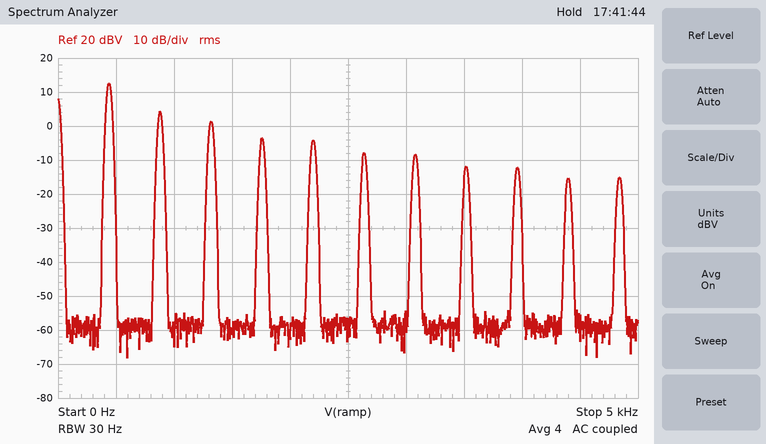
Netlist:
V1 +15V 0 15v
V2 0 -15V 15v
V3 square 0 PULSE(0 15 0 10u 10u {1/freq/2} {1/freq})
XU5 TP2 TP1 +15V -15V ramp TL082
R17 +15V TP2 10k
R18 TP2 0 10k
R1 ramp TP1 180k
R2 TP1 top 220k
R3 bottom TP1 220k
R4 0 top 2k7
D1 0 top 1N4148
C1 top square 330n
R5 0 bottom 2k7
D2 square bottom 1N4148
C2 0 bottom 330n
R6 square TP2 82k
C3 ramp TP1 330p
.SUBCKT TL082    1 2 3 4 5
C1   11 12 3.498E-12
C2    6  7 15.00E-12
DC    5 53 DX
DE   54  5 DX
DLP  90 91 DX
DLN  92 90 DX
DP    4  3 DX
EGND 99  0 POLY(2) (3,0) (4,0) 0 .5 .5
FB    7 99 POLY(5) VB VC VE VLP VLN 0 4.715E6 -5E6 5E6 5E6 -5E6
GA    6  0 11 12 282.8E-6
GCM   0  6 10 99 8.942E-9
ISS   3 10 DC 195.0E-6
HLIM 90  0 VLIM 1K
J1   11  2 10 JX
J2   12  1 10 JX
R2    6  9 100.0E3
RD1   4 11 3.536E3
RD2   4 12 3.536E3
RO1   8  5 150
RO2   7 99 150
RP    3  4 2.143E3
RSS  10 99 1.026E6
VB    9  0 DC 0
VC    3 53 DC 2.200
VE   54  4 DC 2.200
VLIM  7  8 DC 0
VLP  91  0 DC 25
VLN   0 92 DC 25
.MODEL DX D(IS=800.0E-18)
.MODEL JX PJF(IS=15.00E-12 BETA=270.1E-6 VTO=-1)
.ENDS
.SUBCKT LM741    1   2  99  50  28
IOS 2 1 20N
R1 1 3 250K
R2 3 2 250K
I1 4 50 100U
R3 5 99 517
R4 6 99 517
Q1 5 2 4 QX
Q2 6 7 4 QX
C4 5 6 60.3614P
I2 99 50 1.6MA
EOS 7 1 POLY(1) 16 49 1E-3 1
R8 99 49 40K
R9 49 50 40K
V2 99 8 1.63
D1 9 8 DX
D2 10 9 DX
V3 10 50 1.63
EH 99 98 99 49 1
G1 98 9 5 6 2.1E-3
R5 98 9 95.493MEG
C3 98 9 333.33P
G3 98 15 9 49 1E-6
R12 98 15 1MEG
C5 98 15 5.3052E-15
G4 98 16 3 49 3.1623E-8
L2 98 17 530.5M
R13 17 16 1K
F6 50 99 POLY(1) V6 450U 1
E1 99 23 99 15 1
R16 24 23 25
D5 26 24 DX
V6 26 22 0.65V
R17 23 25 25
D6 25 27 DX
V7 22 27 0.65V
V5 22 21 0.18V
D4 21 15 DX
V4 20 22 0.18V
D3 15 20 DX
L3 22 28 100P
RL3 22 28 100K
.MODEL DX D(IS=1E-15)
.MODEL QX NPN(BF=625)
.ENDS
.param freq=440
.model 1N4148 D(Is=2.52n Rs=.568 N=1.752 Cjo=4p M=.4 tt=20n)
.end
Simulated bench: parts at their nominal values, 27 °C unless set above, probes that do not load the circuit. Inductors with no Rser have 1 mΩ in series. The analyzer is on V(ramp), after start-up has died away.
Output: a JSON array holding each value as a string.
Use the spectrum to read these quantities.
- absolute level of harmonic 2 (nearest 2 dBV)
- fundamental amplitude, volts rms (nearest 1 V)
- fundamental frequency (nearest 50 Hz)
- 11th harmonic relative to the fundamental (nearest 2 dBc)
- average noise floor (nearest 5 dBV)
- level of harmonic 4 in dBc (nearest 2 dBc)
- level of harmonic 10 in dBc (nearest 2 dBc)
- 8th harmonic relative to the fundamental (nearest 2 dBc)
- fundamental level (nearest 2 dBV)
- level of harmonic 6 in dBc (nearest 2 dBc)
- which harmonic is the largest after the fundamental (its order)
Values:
["4 dBV", "4 V", "450 Hz", "-28 dBc", "-60 dBV", "-16 dBc", "-28 dBc", "-24 dBc", "12 dBV", "-20 dBc", "2"]
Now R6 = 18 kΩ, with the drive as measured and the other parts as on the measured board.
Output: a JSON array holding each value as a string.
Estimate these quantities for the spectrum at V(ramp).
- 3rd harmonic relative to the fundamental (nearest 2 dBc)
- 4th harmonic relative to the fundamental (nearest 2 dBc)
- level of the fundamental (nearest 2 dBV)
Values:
["-10 dBc", "-6 dBc", "4 dBV"]
